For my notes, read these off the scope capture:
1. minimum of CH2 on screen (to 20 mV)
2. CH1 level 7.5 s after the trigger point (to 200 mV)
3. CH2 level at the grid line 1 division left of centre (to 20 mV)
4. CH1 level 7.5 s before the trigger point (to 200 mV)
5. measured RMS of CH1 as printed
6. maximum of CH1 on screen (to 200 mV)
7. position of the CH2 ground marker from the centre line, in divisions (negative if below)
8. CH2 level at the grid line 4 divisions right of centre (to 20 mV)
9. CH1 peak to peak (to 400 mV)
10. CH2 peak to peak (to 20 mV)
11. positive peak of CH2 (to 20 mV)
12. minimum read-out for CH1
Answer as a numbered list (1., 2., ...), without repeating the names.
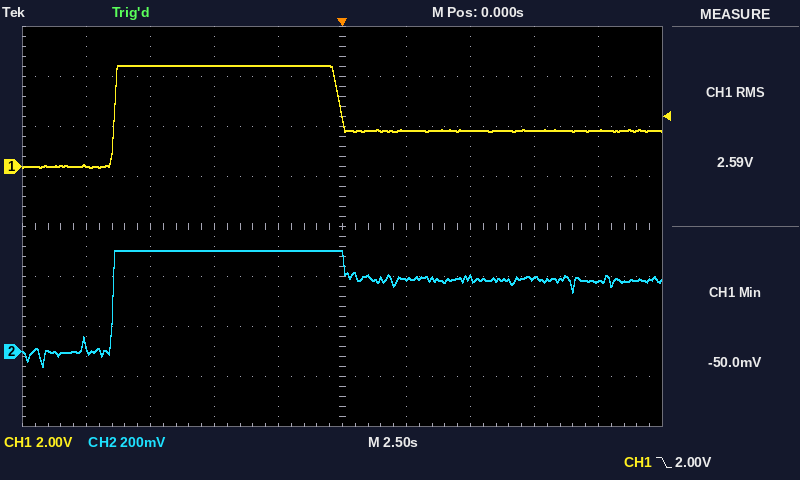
1. -60 mV
2. 1.4 V
3. 400 mV
4. 4.0 V
5. 2.59 V
6. 4.0 V
7. -2.5 div
8. 280 mV
9. 4.0 V
10. 460 mV
11. 400 mV
12. -50.0 mV
